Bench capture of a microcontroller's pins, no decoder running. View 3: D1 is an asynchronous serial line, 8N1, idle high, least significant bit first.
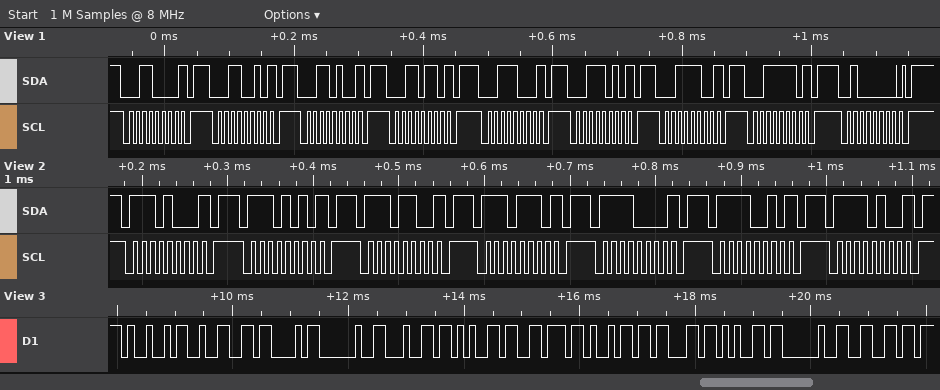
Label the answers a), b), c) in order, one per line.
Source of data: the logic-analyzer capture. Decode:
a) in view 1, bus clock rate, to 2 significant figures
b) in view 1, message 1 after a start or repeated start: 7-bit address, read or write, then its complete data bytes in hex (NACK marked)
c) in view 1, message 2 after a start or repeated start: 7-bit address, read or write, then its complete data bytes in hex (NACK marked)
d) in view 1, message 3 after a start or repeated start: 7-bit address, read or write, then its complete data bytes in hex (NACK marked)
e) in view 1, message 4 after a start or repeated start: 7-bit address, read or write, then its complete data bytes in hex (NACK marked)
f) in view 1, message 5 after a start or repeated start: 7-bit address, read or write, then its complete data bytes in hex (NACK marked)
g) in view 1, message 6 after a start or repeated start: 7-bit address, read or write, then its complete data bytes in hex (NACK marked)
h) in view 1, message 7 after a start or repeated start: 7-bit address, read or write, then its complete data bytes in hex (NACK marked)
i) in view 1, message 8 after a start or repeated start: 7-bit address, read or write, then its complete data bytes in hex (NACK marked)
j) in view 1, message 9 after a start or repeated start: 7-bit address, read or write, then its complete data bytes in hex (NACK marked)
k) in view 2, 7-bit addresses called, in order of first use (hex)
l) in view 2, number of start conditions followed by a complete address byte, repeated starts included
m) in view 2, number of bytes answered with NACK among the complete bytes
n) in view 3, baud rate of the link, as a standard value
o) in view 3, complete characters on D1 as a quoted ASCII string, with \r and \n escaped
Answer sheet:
a) 100 kHz
b) 0x18 write NACK
c) 0x19 write NACK
d) 0x1A write NACK
e) 0x1B write NACK
f) 0x1C write NACK
g) 0x1D write NACK
h) 0x1E write NACK
i) 0x1F write NACK
j) 0x20 write
k) 0x74 0x75 0x76 0x77 0x78 0x79 0x7A
l) 7
m) 7
n) 9600 baud
o) "I2C device f"
